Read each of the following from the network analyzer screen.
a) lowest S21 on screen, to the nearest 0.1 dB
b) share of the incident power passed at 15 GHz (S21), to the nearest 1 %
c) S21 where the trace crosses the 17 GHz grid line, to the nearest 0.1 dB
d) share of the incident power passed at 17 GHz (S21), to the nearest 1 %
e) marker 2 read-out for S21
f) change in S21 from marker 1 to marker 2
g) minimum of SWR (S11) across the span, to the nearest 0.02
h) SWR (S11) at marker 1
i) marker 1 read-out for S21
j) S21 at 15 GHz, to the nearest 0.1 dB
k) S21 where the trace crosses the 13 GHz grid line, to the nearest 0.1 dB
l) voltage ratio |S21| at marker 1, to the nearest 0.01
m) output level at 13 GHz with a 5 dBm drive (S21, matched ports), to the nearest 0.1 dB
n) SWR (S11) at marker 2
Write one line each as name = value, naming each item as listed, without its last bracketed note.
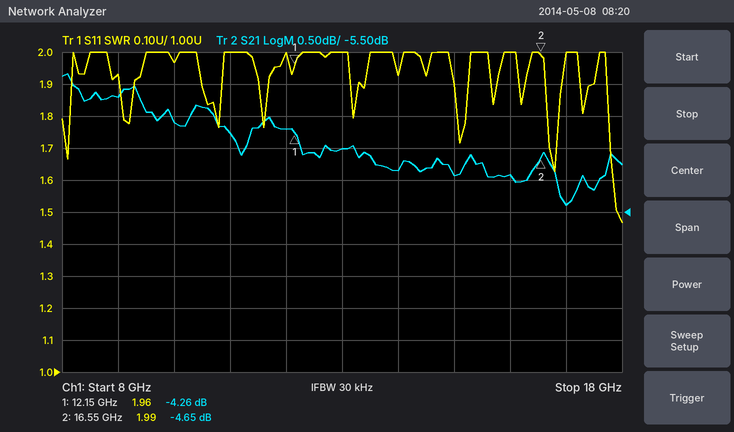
lowest S21 on screen, to the nearest 0.1 dB = -5.4 dB
share of the incident power passed at 15 GHz (S21), to the nearest 1 % = 32 %
S21 where the trace crosses the 17 GHz grid line, to the nearest 0.1 dB = -5.4 dB
share of the incident power passed at 17 GHz (S21), to the nearest 1 % = 29 %
marker 2 read-out for S21 = -4.65 dB
change in S21 from marker 1 to marker 2 = -0.39 dB
minimum of SWR (S11) across the span, to the nearest 0.02 = 1.46
SWR (S11) at marker 1 = 1.96
marker 1 read-out for S21 = -4.26 dB
S21 at 15 GHz, to the nearest 0.1 dB = -4.9 dB
S21 where the trace crosses the 13 GHz grid line, to the nearest 0.1 dB = -4.5 dB
voltage ratio |S21| at marker 1, to the nearest 0.01 = 0.61
output level at 13 GHz with a 5 dBm drive (S21, matched ports), to the nearest 0.1 dB = 0.5 dBm
SWR (S11) at marker 2 = 1.99
